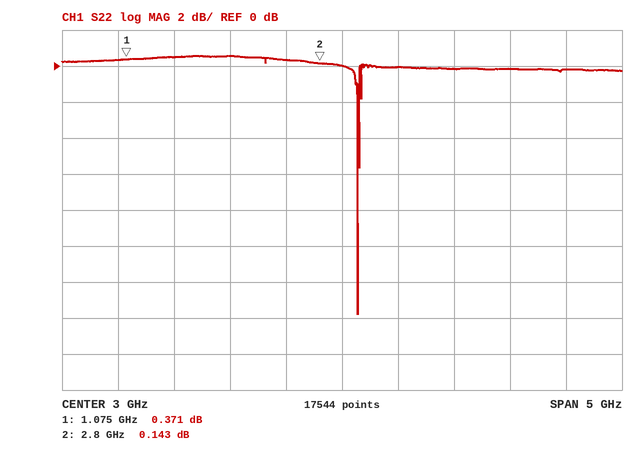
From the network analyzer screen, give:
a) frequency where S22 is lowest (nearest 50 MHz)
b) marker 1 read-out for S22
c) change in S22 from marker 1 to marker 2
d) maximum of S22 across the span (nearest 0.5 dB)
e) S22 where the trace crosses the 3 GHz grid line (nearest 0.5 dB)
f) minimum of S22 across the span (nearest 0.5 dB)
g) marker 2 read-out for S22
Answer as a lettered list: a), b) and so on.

a) 3.15 GHz
b) 0.371 dB
c) -0.228 dB
d) 0.5 dB
e) 0.0 dB
f) -14.0 dB
g) 0.143 dB
